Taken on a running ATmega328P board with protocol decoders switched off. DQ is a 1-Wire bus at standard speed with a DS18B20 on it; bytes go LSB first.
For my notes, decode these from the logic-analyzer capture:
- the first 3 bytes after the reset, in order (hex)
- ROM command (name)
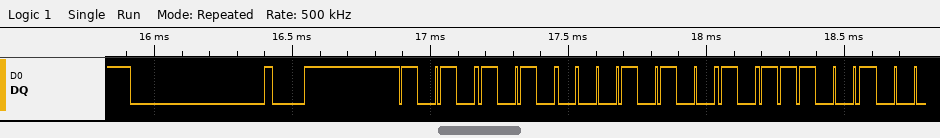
55 28 9D
Match ROM
